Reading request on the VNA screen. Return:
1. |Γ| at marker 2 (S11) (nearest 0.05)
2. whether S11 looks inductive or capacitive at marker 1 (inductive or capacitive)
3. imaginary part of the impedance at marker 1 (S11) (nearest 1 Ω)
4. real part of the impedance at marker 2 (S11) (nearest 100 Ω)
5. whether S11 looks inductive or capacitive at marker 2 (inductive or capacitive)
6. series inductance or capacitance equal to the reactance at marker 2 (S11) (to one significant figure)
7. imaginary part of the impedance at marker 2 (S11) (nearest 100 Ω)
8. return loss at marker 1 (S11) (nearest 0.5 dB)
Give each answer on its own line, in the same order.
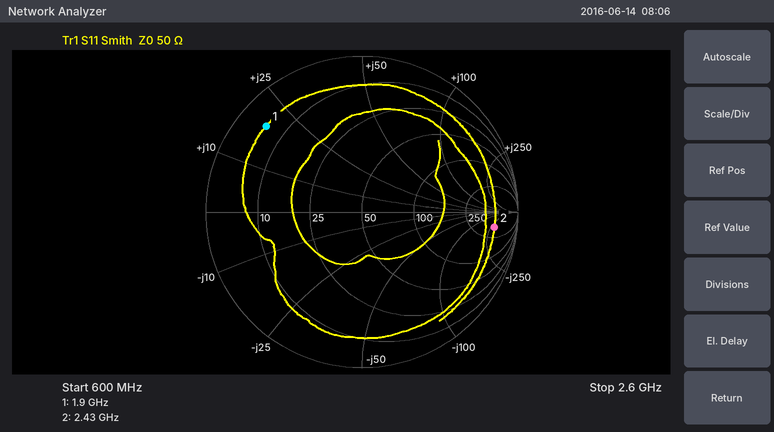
0.85
inductive
+19 Ω
400 Ω
capacitive
200 fF
-300 Ω
1.5 dB
